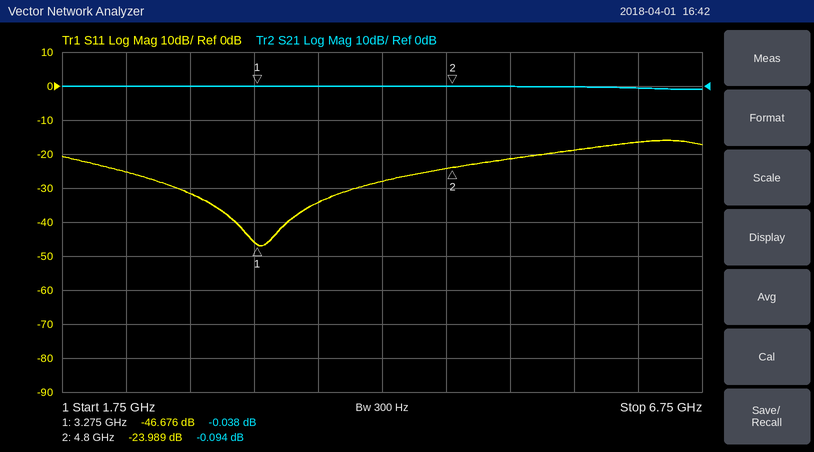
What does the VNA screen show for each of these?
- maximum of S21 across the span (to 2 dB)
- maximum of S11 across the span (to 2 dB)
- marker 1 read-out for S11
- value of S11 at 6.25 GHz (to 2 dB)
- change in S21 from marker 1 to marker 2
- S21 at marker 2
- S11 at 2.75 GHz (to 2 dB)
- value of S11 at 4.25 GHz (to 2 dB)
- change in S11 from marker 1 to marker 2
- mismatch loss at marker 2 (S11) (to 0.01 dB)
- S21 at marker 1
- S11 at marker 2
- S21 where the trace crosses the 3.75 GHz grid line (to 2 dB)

0 dB
-16 dB
-46.676 dB
-16 dB
-0.056 dB
-0.094 dB
-32 dB
-28 dB
22.687 dB
0.02 dB
-0.038 dB
-23.989 dB
0 dB
